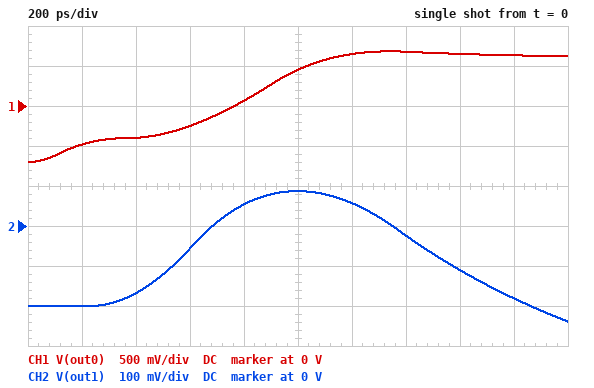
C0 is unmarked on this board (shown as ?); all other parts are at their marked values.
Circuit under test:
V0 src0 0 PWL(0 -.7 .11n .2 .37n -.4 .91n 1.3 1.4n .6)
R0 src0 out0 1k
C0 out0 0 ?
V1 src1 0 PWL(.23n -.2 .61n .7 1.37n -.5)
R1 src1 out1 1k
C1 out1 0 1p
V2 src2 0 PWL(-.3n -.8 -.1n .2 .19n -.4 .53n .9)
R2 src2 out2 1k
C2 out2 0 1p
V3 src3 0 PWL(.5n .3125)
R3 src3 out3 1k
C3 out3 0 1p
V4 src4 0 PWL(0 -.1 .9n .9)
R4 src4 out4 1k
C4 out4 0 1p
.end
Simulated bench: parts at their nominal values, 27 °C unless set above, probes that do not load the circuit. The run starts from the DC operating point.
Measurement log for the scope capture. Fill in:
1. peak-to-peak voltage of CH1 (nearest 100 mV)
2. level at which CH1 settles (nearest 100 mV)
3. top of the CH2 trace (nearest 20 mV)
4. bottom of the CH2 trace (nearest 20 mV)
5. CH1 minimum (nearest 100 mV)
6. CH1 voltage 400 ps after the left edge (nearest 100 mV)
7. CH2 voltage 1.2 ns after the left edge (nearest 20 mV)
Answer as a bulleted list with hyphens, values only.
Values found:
- 1.4 V
- 600 mV
- 80 mV
- -240 mV
- -700 mV
- -400 mV
- 60 mV
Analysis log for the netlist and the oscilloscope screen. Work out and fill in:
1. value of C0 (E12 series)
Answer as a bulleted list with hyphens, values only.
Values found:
- 470 fF
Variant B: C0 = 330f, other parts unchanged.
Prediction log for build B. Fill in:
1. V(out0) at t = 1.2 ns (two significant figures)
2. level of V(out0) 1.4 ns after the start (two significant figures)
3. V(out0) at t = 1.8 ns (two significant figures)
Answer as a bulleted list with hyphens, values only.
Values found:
- 820 mV
- 780 mV
- 650 mV
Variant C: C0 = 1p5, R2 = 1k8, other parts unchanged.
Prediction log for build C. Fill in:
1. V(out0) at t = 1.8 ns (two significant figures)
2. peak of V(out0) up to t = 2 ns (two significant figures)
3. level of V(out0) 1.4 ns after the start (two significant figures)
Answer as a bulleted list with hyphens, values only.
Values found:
- 200 mV
- 250 mV
- 77 mV
